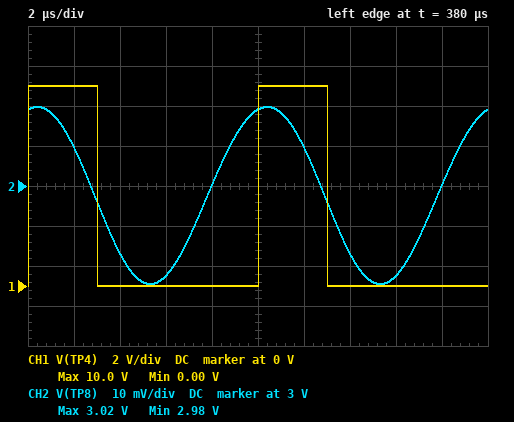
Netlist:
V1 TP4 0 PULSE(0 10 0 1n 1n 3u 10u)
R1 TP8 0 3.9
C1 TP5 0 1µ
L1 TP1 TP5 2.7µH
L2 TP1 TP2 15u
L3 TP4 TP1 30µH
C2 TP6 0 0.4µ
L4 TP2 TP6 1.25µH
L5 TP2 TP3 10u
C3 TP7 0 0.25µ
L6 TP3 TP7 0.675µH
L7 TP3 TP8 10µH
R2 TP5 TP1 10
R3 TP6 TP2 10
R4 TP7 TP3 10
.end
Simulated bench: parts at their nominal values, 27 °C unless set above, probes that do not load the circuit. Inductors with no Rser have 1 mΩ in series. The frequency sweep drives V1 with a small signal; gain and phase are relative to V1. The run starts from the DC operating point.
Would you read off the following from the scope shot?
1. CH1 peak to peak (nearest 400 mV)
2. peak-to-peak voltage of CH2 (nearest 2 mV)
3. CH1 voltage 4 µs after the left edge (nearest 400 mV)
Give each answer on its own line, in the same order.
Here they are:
10.0 V
44 mV
0 V
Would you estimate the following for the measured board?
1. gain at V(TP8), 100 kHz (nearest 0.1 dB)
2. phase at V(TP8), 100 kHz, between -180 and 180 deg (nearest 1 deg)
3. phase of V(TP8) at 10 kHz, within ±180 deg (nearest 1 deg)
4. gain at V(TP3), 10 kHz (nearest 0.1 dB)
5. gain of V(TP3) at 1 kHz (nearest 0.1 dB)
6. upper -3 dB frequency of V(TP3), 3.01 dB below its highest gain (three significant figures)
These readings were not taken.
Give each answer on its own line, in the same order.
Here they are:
-47.3 dB
41 deg
-51 deg
-1.6 dB
0 dB
37.3 kHz
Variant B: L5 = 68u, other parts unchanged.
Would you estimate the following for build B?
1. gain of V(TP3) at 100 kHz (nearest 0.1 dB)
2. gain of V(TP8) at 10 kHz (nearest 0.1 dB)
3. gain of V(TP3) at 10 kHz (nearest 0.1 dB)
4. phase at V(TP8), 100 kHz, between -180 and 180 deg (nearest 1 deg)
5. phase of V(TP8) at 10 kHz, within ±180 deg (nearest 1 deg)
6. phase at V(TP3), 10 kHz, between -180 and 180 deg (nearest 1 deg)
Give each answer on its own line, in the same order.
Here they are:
-51.6 dB
-5.3 dB
-5.2 dB
-62 deg
-67 deg
-58 deg
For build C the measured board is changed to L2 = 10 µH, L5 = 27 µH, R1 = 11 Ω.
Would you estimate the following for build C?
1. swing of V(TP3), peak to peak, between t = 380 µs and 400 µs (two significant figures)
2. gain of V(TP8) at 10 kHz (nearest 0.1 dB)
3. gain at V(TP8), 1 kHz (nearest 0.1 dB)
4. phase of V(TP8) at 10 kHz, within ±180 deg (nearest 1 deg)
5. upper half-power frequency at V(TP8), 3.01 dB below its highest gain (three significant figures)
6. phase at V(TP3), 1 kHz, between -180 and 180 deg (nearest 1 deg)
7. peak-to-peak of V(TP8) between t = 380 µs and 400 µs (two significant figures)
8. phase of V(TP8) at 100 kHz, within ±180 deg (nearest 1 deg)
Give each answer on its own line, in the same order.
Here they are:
180 mV
1.4 dB
0 dB
-27 deg
29.1 kHz
-2 deg
160 mV
-32 deg
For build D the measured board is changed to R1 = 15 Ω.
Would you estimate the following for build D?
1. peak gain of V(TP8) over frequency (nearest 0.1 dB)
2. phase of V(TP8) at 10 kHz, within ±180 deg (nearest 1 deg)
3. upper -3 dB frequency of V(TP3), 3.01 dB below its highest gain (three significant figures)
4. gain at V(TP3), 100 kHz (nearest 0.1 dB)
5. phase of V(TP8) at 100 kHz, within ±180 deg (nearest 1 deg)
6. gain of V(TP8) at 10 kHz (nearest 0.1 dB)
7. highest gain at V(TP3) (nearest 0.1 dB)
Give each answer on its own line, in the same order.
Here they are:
9.3 dB
-18 deg
25.7 kHz
-40.4 dB
76 deg
1.9 dB
9.4 dB
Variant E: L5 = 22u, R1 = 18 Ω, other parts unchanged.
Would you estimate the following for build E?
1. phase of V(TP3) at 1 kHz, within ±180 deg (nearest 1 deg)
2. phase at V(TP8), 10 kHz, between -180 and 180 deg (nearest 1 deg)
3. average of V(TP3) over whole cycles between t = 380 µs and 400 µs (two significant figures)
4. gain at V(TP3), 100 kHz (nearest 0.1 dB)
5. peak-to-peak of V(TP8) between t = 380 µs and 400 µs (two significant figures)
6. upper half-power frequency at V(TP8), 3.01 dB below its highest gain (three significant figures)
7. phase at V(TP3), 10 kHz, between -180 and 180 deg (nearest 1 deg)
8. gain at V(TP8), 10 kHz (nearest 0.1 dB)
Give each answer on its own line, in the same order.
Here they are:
-1 deg
-18 deg
3.0 V
-37.8 dB
130 mV
25.5 kHz
-16 deg
2.1 dB
